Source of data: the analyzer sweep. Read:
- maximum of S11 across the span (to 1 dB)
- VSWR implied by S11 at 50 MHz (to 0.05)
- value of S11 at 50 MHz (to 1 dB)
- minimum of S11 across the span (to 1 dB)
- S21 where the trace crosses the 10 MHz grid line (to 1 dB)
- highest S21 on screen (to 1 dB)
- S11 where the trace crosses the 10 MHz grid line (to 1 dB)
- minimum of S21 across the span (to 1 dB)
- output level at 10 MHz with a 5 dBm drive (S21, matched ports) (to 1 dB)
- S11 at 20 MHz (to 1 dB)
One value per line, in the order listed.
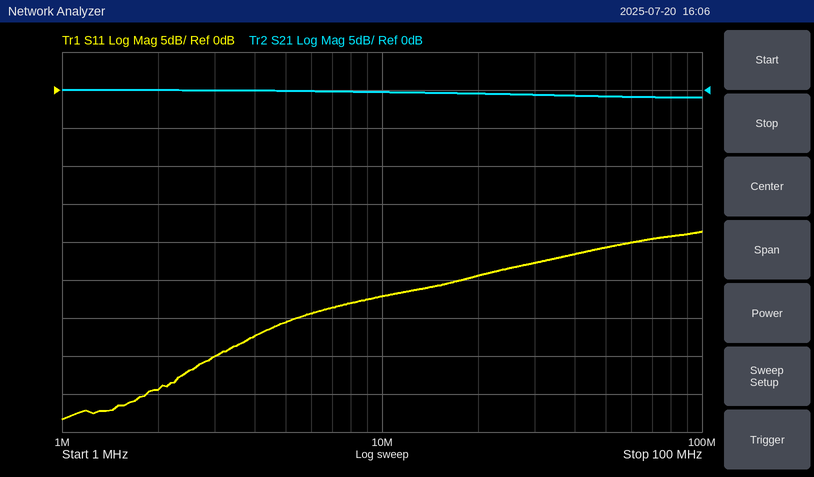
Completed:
-19 dB
1.20
-21 dB
-43 dB
0 dB
0 dB
-27 dB
-1 dB
5 dBm
-24 dB
